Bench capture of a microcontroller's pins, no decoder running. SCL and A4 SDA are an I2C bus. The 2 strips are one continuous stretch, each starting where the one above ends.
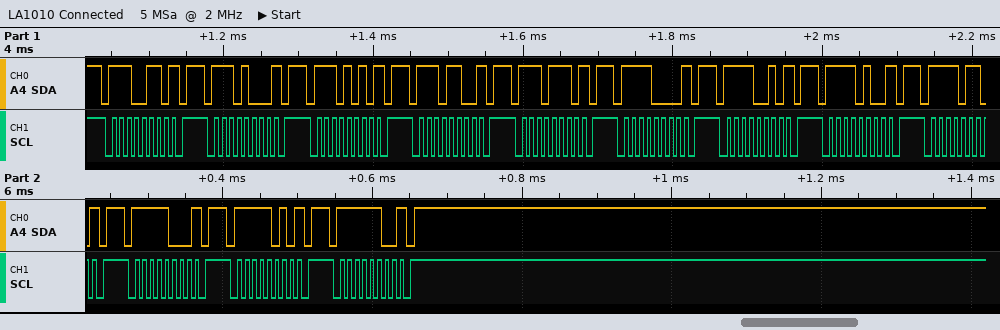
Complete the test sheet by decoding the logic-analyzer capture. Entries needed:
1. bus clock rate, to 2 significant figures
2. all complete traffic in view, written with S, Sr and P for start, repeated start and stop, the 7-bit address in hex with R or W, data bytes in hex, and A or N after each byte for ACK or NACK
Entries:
100 kHz
S 73W N P S 74W N P S 75W N P S 76W N P S 77W N P S 78W N P S 79W N P S 7AW N P S 7BW N P S 7CW N P S 7DW N P S 7EW N P
